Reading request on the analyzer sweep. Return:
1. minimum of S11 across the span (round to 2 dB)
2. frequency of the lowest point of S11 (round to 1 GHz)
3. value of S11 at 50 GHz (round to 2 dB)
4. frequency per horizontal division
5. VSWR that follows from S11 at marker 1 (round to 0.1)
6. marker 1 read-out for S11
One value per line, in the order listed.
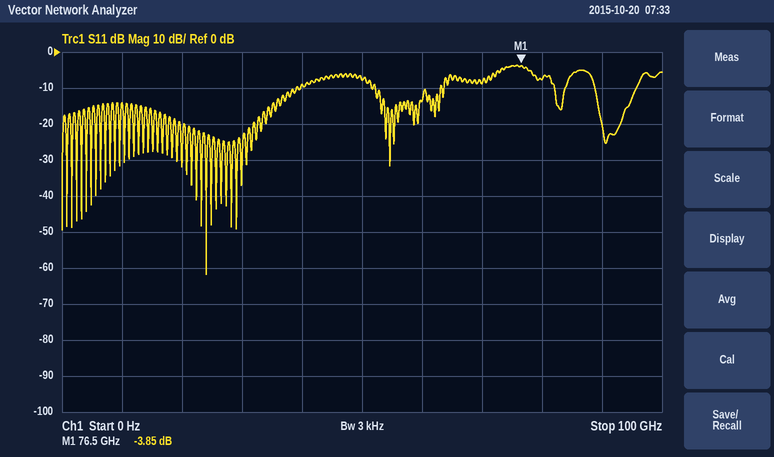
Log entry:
-62 dB
24 GHz
-8 dB
10 GHz
4.6
-3.85 dB
